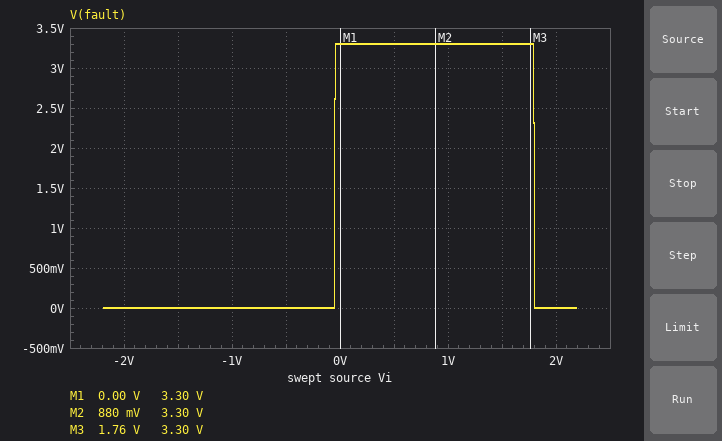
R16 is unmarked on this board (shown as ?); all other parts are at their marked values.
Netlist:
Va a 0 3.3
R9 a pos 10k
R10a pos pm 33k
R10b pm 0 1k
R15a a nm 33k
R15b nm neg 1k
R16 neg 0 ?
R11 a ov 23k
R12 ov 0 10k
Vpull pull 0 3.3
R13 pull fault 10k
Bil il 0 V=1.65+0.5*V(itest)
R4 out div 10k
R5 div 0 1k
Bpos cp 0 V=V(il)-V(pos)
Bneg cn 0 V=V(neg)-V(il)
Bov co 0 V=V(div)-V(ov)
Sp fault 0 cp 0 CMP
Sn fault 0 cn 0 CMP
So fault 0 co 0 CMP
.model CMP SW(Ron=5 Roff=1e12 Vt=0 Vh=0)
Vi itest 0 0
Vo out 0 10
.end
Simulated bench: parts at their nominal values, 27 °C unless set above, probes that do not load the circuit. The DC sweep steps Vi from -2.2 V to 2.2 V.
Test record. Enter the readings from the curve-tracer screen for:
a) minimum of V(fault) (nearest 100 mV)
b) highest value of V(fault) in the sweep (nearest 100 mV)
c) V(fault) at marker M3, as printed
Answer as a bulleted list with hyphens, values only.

- 0 V
- 3.3 V
- 3.30 V
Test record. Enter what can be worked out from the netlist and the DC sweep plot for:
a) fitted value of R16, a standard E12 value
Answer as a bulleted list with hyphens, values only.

- 33 kΩ
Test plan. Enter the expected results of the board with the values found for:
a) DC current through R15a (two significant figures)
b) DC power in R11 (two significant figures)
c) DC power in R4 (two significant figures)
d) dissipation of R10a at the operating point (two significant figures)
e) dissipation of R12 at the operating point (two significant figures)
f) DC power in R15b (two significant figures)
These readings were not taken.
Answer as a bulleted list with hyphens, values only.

- 49 µA
- 230 µW
- 8.3 mW
- 190 µW
- 100 µW
- 2.4 µW
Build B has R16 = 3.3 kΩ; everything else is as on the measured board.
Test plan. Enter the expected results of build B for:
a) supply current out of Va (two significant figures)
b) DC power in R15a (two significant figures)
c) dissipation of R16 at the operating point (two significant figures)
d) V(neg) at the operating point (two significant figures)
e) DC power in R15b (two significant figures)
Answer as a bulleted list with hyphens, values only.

- 260 µA
- 260 µW
- 26 µW
- 290 mV
- 7.8 µW
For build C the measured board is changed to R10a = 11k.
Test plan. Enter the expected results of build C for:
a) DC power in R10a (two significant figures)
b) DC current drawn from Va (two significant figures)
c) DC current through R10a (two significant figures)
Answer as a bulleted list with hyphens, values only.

- 250 µW
- 300 µA
- 150 µA
